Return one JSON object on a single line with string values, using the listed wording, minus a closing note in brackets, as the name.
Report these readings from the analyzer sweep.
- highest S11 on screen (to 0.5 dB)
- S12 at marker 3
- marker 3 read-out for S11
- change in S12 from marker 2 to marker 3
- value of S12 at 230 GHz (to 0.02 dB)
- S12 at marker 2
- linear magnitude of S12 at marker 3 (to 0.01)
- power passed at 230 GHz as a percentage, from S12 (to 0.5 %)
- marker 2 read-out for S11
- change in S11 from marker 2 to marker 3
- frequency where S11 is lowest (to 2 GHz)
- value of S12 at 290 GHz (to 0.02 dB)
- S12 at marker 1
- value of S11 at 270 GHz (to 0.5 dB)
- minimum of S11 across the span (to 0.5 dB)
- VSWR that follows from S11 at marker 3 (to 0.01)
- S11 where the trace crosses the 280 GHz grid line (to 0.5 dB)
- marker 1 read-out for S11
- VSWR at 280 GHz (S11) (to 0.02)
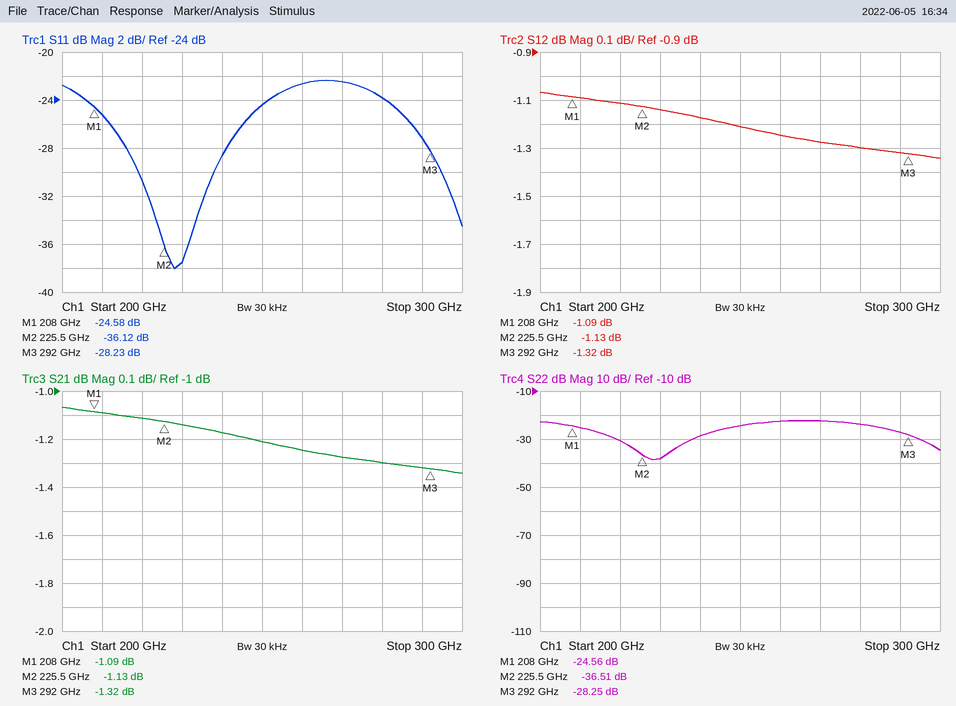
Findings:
{"highest S11 on screen": "-22.5 dB", "S12 at marker 3": "-1.32 dB", "marker 3 read-out for S11": "-28.23 dB", "change in S12 from marker 2 to marker 3": "-0.19 dB", "value of S12 at 230 GHz": "-1.14 dB", "S12 at marker 2": "-1.13 dB", "linear magnitude of S12 at marker 3": "0.86", "power passed at 230 GHz as a percentage, from S12": "77.0 %", "marker 2 read-out for S11": "-36.12 dB", "change in S11 from marker 2 to marker 3": "7.89 dB", "frequency where S11 is lowest": "228 GHz", "value of S12 at 290 GHz": "-1.32 dB", "S12 at marker 1": "-1.09 dB", "value of S11 at 270 GHz": "-22.5 dB", "minimum of S11 across the span": "-38.0 dB", "VSWR that follows from S11 at marker 3": "1.08", "S11 where the trace crosses the 280 GHz grid line": "-24.0 dB", "marker 1 read-out for S11": "-24.58 dB", "VSWR at 280 GHz (S11)": "1.14"}
